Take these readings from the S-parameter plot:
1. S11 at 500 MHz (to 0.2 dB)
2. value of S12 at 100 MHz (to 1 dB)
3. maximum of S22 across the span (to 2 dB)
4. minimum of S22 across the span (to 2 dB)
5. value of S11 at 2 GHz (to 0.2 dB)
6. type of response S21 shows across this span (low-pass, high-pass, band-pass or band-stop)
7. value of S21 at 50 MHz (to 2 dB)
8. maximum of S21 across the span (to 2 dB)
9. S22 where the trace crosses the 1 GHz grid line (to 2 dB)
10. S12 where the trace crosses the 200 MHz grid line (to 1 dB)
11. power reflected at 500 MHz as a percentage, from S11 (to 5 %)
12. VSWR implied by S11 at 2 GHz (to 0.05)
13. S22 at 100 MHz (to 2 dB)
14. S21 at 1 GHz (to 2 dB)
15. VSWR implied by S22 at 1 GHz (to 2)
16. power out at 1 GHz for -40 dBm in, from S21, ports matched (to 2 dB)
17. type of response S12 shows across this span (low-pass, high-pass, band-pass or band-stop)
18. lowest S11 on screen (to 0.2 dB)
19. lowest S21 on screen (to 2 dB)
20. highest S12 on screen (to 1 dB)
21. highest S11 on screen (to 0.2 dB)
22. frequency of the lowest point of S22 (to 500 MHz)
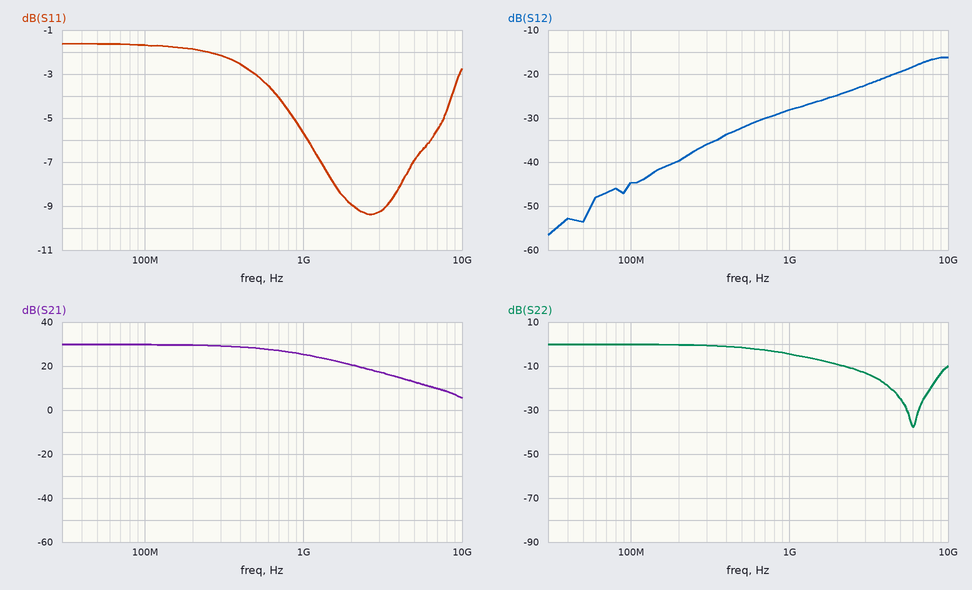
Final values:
-3.0 dB
-45 dB
0 dB
-38 dB
-9.0 dB
low-pass
30 dB
30 dB
-4 dB
-40 dB
50 %
2.10
0 dB
26 dB
4
-14 dBm
high-pass
-9.4 dB
6 dB
-16 dB
-1.6 dB
6.0 GHz
